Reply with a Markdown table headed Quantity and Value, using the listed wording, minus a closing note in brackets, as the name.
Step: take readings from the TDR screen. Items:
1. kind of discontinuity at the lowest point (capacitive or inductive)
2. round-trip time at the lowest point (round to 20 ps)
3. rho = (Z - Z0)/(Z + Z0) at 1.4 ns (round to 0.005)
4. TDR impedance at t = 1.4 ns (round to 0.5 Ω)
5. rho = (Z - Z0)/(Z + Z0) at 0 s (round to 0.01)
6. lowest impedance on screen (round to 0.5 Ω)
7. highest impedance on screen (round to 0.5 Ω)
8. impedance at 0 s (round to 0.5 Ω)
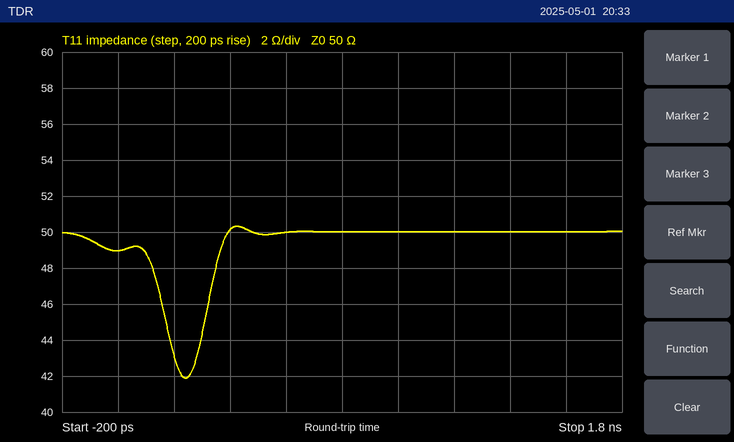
| Quantity | Value |
|---|---|
| kind of discontinuity at the lowest point | capacitive |
| round-trip time at the lowest point | 240 ps |
| rho = (Z - Z0)/(Z + Z0) at 1.4 ns | 0.000 |
| TDR impedance at t = 1.4 ns | 50.0 Ω |
| rho = (Z - Z0)/(Z + Z0) at 0 s | -0.01 |
| lowest impedance on screen | 42.0 Ω |
| highest impedance on screen | 50.5 Ω |
| impedance at 0 s | 49.0 Ω |
